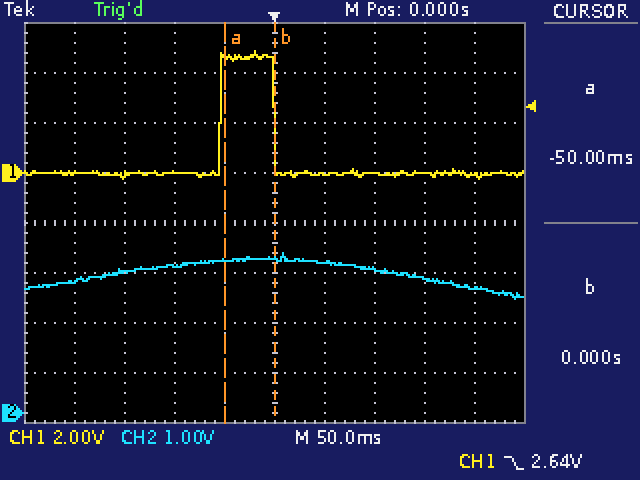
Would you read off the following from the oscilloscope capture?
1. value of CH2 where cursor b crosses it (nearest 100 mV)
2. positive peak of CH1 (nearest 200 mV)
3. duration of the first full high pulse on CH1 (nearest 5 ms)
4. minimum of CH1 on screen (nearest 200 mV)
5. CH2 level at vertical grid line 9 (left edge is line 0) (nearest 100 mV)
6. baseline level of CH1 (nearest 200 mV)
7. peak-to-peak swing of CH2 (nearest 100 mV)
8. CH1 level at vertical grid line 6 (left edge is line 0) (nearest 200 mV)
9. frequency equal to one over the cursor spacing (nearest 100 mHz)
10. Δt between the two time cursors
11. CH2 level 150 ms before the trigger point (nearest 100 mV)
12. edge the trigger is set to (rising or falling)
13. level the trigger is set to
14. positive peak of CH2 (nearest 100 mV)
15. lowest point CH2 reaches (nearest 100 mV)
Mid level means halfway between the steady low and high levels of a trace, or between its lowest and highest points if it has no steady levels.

3.1 V
4.8 V
55 ms
-200 mV
2.5 V
0.0 V
900 mV
0.0 V
20.0 Hz
50 ms
2.8 V
falling
2.64 V
3.2 V
2.3 V
